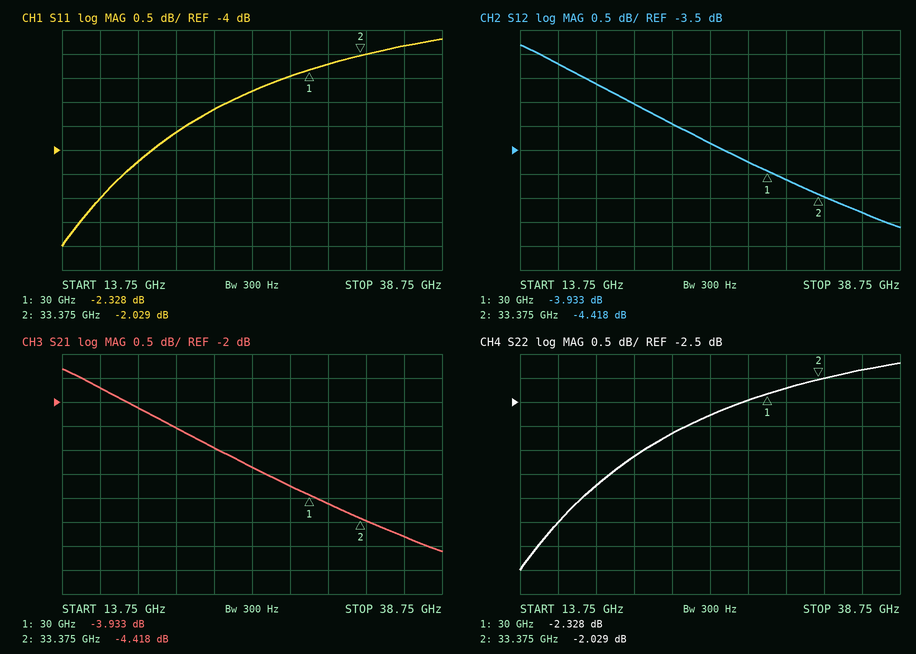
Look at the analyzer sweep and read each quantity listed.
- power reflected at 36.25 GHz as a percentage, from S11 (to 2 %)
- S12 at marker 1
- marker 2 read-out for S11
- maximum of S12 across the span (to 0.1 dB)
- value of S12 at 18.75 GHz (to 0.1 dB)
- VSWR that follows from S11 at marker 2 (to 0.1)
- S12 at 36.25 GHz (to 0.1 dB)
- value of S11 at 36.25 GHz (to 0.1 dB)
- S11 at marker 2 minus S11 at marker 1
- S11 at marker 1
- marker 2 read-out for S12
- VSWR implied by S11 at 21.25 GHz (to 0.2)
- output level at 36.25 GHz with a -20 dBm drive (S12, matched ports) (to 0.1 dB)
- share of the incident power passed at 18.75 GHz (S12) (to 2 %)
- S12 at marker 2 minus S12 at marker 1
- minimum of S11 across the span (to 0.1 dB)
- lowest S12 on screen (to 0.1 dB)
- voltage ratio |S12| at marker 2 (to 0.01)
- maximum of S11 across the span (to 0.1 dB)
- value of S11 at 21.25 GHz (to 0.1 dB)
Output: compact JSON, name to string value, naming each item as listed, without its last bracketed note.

{"power reflected at 36.25 GHz as a percentage, from S11": "66 %", "S12 at marker 1": "-3.933 dB", "marker 2 read-out for S11": "-2.029 dB", "maximum of S12 across the span": "-1.3 dB", "value of S12 at 18.75 GHz": "-2.1 dB", "VSWR that follows from S11 at marker 2": "8.6", "S12 at 36.25 GHz": "-4.8 dB", "value of S11 at 36.25 GHz": "-1.8 dB", "S11 at marker 2 minus S11 at marker 1": "0.299 dB", "S11 at marker 1": "-2.328 dB", "marker 2 read-out for S12": "-4.418 dB", "VSWR implied by S11 at 21.25 GHz": "4.8", "output level at 36.25 GHz with a -20 dBm drive (S12, matched ports)": "-24.8 dBm", "share of the incident power passed at 18.75 GHz (S12)": "62 %", "S12 at marker 2 minus S12 at marker 1": "-0.485 dB", "minimum of S11 across the span": "-6.0 dB", "lowest S12 on screen": "-5.1 dB", "voltage ratio |S12| at marker 2": "0.60", "maximum of S11 across the span": "-1.7 dB", "value of S11 at 21.25 GHz": "-3.6 dB"}
